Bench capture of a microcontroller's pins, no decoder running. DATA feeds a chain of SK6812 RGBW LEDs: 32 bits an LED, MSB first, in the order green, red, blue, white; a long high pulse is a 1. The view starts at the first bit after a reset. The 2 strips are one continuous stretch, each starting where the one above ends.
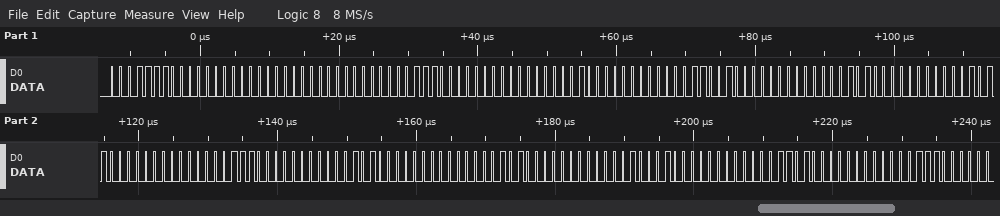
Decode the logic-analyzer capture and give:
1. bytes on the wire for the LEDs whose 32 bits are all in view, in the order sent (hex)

1E 00 00 00 1C 00 02 00 19 00 05 00 16 00 07 00 14 00 0A 00 11 00 0D 00
